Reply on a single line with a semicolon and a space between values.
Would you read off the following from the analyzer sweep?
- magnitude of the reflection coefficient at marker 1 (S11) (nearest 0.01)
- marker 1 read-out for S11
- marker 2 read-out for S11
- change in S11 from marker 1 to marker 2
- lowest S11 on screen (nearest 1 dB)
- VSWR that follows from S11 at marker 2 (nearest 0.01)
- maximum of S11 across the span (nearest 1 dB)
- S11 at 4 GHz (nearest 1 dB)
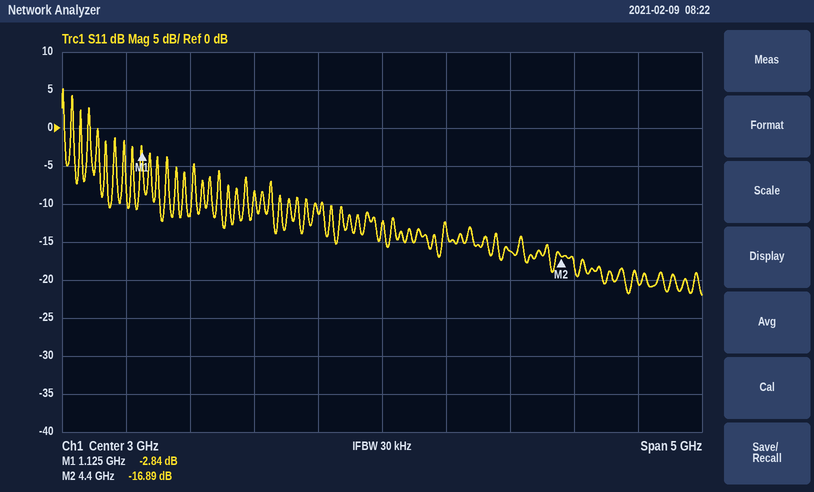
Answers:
0.72; -2.84 dB; -16.89 dB; -14.05 dB; -22 dB; 1.33; 5 dB; -16 dB
